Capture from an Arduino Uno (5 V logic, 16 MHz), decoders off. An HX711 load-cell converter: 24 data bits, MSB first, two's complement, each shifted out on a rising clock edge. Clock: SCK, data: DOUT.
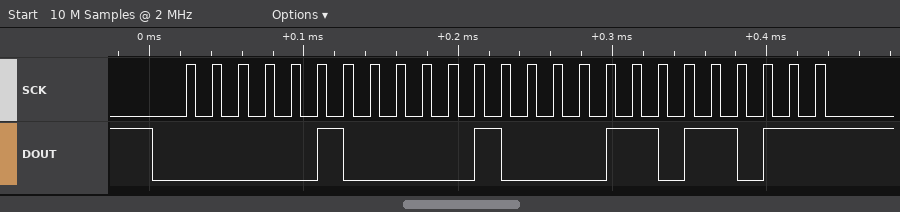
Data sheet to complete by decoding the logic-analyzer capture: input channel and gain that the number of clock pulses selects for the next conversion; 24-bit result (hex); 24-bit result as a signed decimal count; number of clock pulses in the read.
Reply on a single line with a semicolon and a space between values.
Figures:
channel A, gain 128; 0x0410DB; 266459; 25
